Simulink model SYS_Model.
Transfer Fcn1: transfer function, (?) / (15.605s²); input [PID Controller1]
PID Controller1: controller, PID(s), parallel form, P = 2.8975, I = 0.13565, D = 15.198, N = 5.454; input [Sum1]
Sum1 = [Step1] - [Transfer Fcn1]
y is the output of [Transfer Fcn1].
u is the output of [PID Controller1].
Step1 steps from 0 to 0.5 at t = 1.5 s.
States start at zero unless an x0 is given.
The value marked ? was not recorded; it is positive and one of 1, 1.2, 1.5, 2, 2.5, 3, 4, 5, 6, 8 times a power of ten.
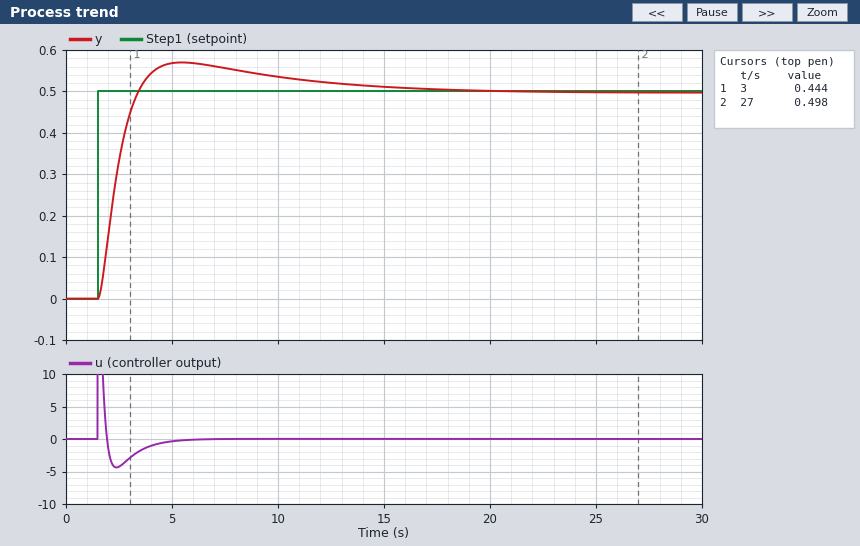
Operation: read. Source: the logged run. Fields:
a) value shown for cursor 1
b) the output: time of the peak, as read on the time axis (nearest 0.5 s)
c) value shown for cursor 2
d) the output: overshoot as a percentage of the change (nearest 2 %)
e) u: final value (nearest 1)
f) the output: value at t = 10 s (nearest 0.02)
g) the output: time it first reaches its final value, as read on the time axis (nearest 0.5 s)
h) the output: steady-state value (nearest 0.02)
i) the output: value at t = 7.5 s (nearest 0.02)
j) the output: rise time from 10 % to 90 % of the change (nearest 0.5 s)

0.444
5.5 s
0.498
14 %
0
0.54
3.5 s
0.50
0.56
1.5 s
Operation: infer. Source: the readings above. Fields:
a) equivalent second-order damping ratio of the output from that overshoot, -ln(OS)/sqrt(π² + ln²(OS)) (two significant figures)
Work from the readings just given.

0.53
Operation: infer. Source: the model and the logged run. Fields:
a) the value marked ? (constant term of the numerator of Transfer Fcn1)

1
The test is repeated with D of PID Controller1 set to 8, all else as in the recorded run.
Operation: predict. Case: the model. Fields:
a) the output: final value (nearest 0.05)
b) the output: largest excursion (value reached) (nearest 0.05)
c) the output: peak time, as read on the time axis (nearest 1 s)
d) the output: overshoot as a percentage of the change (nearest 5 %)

0.50
0.65
7 s
30 %
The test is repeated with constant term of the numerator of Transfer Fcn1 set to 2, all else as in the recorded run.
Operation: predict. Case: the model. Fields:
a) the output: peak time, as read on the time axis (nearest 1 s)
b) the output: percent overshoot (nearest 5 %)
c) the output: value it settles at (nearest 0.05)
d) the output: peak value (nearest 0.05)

3 s
10 %
0.50
0.55
